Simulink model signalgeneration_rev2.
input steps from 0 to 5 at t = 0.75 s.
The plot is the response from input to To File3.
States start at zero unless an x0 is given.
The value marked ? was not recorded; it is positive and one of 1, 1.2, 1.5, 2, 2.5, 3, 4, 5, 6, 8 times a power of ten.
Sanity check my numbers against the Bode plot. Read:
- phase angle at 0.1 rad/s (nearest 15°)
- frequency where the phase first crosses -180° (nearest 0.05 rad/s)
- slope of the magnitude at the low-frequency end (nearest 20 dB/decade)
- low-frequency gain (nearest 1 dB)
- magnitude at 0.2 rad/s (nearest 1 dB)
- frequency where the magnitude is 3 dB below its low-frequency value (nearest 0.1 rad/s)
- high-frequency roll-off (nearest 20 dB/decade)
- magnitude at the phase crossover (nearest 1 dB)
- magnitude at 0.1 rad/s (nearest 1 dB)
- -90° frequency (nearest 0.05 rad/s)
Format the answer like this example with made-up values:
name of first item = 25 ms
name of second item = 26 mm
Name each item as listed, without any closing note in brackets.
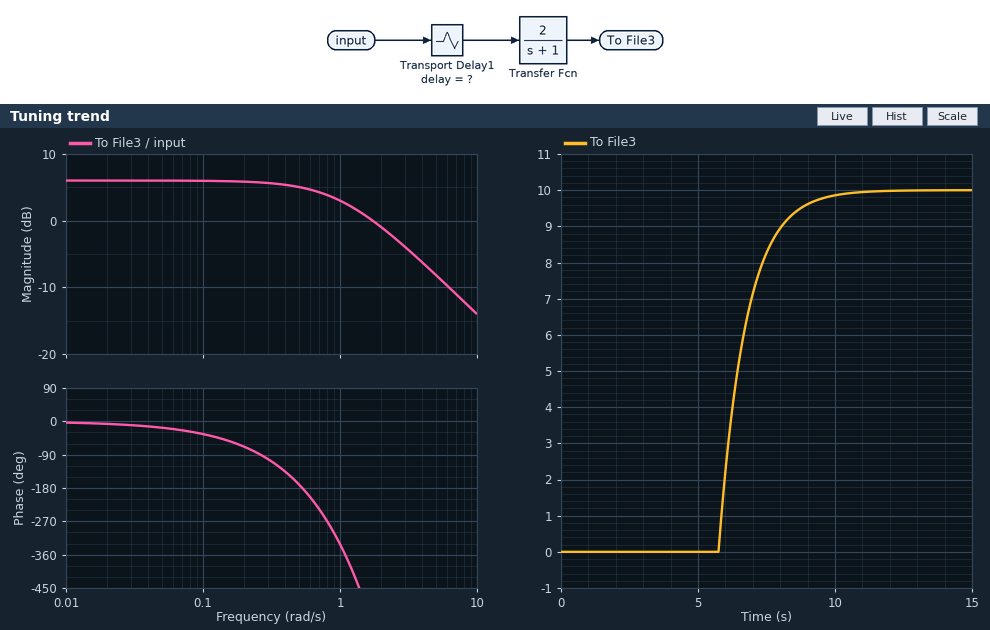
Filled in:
phase angle at 0.1 rad/s = -30°
frequency where the phase first crosses -180° = 0.55 rad/s
slope of the magnitude at the low-frequency end = 0 dB/decade
low-frequency gain = 6 dB
magnitude at 0.2 rad/s = 6 dB
frequency where the magnitude is 3 dB below its low-frequency value = 1.0 rad/s
high-frequency roll-off = -20 dB/decade
magnitude at the phase crossover = 5 dB
magnitude at 0.1 rad/s = 6 dB
-90° frequency = 0.25 rad/s
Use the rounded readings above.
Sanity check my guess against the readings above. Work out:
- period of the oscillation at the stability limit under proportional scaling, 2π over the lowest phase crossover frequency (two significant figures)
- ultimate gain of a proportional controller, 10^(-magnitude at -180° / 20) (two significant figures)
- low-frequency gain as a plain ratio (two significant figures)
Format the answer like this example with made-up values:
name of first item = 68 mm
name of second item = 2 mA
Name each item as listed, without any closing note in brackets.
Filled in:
period of the oscillation at the stability limit under proportional scaling, 2π over the lowest phase crossover frequency = 11 s
ultimate gain of a proportional controller, 10^(-magnitude at -180° / 20) = 0.56
low-frequency gain as a plain ratio = 2.0
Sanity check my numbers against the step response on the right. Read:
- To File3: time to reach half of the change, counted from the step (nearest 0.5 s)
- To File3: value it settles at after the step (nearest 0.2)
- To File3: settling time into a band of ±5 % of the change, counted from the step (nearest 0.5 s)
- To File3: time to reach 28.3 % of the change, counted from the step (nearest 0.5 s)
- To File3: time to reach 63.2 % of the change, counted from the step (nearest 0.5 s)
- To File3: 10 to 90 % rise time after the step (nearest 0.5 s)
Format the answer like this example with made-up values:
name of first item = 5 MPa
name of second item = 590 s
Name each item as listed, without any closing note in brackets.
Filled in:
To File3: time to reach half of the change, counted from the step = 5.5 s
To File3: value it settles at after the step = 10.0
To File3: settling time into a band of ±5 % of the change, counted from the step = 8.0 s
To File3: time to reach 28.3 % of the change, counted from the step = 5.5 s
To File3: time to reach 63.2 % of the change, counted from the step = 6.0 s
To File3: 10 to 90 % rise time after the step = 2.0 s
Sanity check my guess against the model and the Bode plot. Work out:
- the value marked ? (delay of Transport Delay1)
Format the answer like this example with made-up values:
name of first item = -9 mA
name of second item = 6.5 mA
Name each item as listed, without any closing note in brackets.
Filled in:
the value marked ? = 5
